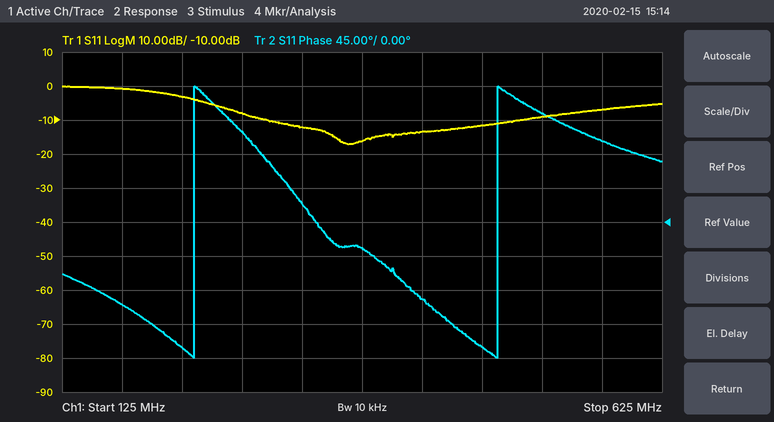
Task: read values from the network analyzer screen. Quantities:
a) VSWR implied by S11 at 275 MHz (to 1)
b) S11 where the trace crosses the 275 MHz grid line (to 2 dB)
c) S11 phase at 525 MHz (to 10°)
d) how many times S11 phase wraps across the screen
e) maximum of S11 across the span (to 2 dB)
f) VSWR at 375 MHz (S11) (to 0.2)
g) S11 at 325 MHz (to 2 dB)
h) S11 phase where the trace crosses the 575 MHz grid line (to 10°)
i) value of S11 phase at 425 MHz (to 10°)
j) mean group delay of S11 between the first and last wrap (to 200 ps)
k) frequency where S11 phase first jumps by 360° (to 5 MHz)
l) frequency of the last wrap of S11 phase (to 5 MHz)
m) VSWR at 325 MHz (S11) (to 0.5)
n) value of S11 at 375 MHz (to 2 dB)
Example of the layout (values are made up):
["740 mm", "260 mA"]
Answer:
["2", "-8 dB", "140°", "2", "0 dB", "1.4", "-12 dB", "110°", "-100°", "4.0 ns", "235 MHz", "490 MHz", "1.5", "-16 dB"]
